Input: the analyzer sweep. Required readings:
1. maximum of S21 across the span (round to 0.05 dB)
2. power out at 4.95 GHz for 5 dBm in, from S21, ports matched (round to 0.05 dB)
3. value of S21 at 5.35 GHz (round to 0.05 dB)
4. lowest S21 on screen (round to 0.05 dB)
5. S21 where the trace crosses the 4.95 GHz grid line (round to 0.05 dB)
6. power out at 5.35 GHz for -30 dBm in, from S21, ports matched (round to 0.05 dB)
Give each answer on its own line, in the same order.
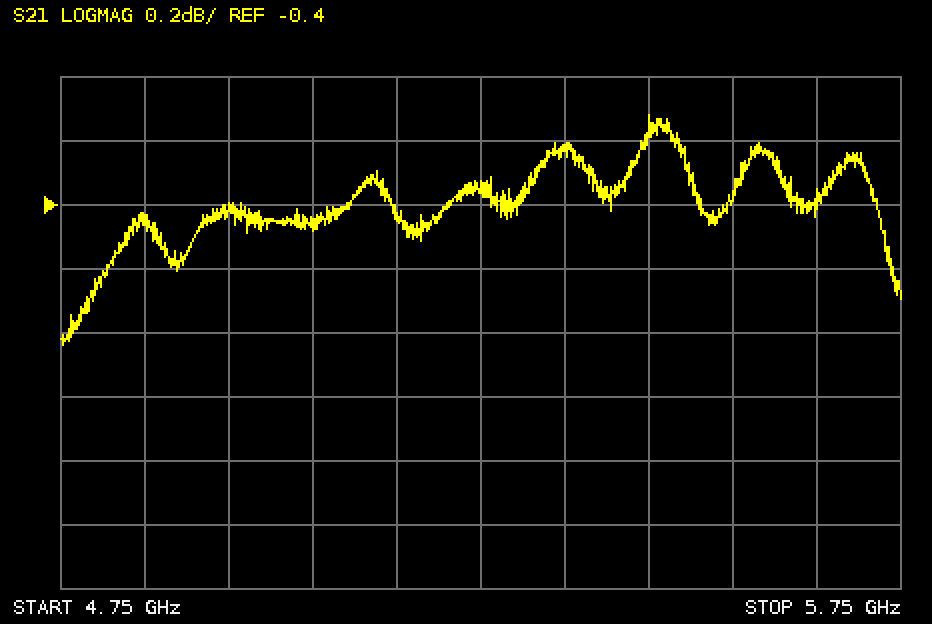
-0.10 dB
4.60 dBm
-0.20 dB
-0.85 dB
-0.40 dB
-30.20 dBm
